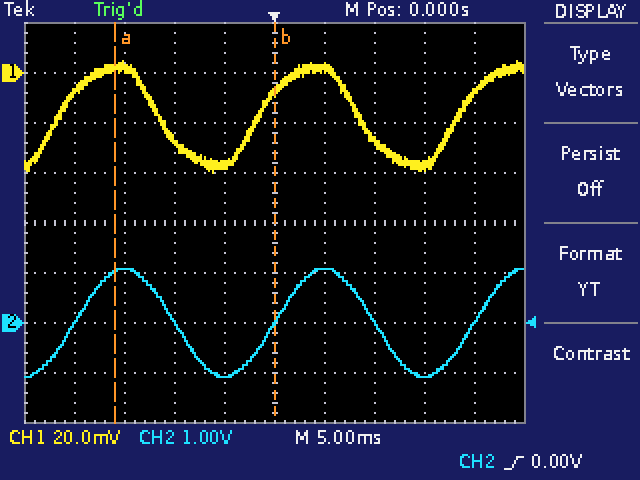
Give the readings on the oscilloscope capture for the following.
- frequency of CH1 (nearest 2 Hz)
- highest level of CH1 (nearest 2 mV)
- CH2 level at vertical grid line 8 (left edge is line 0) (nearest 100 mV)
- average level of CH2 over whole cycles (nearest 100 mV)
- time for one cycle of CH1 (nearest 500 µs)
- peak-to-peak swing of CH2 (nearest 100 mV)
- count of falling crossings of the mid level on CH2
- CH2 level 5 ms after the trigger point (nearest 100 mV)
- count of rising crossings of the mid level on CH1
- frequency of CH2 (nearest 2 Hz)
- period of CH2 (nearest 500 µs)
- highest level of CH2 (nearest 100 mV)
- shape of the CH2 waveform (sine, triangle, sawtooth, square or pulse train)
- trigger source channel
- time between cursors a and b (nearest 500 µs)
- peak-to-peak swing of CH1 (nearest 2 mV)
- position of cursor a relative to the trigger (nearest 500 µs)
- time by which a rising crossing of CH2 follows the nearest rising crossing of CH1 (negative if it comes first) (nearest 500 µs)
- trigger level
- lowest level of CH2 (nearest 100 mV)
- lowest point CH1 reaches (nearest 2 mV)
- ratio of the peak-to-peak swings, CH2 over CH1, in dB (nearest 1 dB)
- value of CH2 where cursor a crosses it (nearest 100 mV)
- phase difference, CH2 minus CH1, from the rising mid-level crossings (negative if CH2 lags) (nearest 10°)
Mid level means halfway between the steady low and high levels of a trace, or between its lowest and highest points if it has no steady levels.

50 Hz
4 mV
-1.1 V
0.0 V
20.0 ms
2.2 V
2
1.1 V
3
50 Hz
20.0 ms
1.1 V
sine
CH2
16.0 ms
44 mV
-16.0 ms
+1.5 ms
0.00 V
-1.1 V
-40 mV
34 dB
1.0 V
-30°
